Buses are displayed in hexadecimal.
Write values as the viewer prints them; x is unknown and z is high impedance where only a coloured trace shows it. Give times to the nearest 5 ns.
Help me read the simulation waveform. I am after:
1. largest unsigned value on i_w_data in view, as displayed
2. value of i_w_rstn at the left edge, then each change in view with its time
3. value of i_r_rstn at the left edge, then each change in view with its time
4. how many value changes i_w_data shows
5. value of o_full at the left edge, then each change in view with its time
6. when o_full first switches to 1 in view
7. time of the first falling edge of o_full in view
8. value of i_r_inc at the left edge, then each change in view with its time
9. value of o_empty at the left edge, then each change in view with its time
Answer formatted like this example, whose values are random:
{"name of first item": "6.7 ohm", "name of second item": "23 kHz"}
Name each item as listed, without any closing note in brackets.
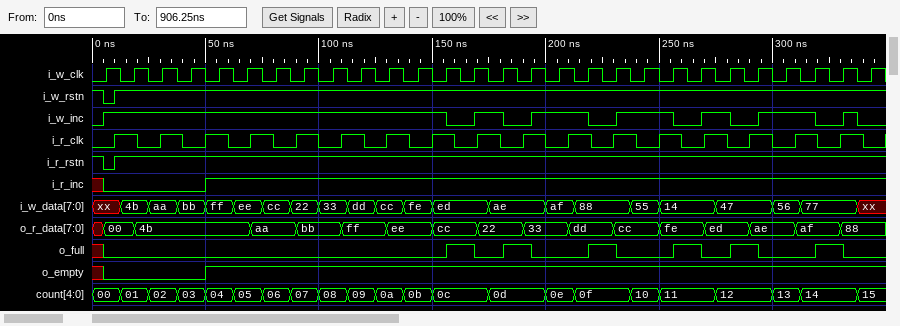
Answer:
{"largest unsigned value on i_w_data in view, as displayed": "ff", "value of i_w_rstn at the left edge, then each change in view with its time": "1, 0 at 5 ns, 1 at 10 ns", "value of i_r_rstn at the left edge, then each change in view with its time": "1, 0 at 5 ns, 1 at 10 ns", "how many value changes i_w_data shows": "21", "value of o_full at the left edge, then each change in view with its time": "x, 0 at 5 ns, 1 at 155 ns, 0 at 170 ns, 1 at 180 ns, 0 at 195 ns, 1 at 220 ns, 0 at 230 ns, 1 at 255 ns, 0 at 270 ns, 1 at 280 ns, 0 at 295 ns, 1 at 320 ns, 0 at 330 ns", "when o_full first switches to 1 in view": "155 ns", "time of the first falling edge of o_full in view": "170 ns", "value of i_r_inc at the left edge, then each change in view with its time": "x, 0 at 5 ns, 1 at 50 ns", "value of o_empty at the left edge, then each change in view with its time": "x, 0 at 5 ns, 1 at 50 ns"}
